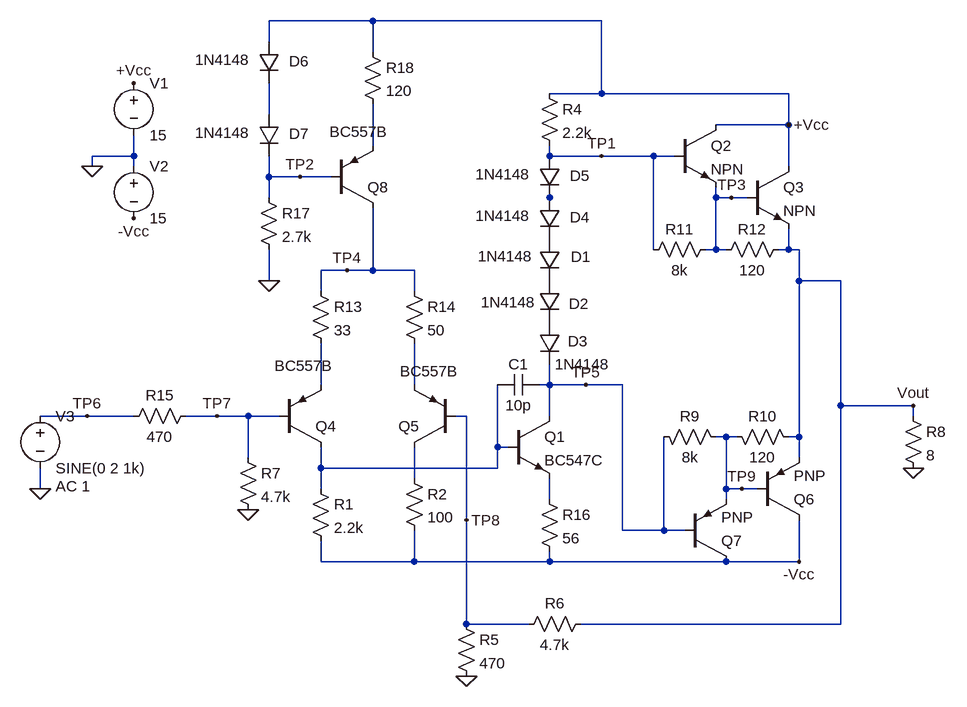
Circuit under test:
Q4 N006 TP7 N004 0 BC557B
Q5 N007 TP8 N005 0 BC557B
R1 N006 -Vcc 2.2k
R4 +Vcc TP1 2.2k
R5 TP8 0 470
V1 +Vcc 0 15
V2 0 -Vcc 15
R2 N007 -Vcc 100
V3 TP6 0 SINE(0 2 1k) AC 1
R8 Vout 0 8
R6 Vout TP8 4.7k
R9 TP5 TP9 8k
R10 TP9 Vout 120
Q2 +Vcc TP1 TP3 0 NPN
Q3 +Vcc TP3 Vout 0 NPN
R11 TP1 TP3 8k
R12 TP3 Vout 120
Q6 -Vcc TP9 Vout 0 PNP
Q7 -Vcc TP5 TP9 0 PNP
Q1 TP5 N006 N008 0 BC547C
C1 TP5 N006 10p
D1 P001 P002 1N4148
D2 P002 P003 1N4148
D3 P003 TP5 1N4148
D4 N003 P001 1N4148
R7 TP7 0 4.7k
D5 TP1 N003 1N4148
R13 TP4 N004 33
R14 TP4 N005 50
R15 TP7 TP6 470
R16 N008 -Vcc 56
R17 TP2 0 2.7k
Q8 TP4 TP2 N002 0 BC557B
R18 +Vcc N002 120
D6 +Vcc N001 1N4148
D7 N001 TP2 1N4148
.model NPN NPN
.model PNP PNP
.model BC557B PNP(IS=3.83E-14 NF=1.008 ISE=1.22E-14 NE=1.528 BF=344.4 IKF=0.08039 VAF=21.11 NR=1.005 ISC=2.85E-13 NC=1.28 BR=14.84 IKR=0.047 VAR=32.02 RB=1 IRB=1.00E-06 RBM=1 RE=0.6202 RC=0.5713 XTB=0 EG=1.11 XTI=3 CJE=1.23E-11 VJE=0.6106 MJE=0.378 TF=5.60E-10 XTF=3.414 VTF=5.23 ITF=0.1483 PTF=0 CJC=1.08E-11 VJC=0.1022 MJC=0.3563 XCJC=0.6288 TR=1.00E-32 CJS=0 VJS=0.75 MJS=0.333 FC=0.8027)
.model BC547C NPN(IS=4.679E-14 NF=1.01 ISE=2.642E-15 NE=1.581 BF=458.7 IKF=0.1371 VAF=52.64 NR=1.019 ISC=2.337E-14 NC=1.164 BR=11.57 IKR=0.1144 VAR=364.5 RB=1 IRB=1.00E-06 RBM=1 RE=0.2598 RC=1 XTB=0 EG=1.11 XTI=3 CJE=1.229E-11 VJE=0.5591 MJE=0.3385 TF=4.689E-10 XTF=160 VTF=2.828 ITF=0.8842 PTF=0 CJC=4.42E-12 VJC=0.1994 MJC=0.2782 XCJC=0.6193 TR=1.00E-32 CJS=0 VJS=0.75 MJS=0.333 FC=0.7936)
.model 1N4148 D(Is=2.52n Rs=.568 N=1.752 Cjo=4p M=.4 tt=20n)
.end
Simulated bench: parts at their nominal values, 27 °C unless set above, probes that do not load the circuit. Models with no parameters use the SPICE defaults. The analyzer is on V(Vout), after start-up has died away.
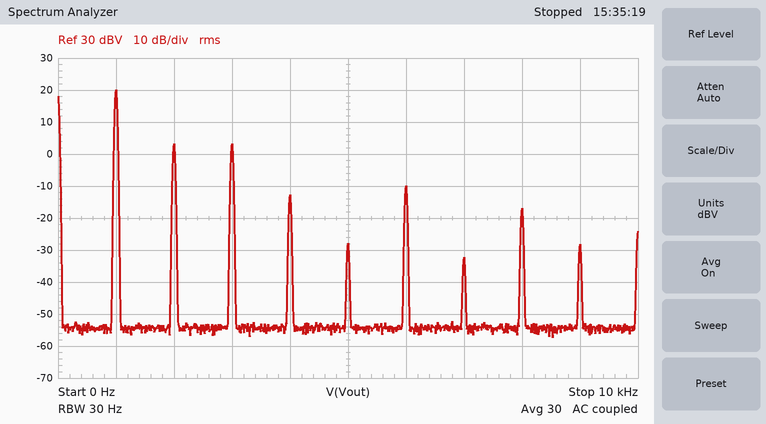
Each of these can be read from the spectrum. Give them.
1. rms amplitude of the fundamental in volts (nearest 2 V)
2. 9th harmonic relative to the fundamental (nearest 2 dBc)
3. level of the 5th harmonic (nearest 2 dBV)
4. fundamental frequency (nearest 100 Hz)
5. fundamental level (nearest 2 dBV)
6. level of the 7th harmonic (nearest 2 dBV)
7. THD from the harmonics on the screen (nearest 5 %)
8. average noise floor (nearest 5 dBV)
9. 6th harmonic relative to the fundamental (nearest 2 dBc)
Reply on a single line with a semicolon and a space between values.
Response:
10 V; -48 dBc; -28 dBV; 1.0 kHz; 20 dBV; -32 dBV; 20 %; -55 dBV; -30 dBc
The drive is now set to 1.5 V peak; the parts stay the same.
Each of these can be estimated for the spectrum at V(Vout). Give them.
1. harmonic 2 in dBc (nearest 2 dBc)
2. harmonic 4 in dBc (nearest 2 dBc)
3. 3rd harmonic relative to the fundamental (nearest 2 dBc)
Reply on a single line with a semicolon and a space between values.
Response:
-18 dBc; -30 dBc; -22 dBc
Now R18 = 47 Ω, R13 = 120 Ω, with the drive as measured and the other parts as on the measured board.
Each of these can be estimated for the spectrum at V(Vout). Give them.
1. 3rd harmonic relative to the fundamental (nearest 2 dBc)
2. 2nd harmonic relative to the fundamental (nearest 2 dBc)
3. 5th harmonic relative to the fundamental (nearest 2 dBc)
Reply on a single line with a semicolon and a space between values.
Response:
-22 dBc; -10 dBc; -28 dBc
